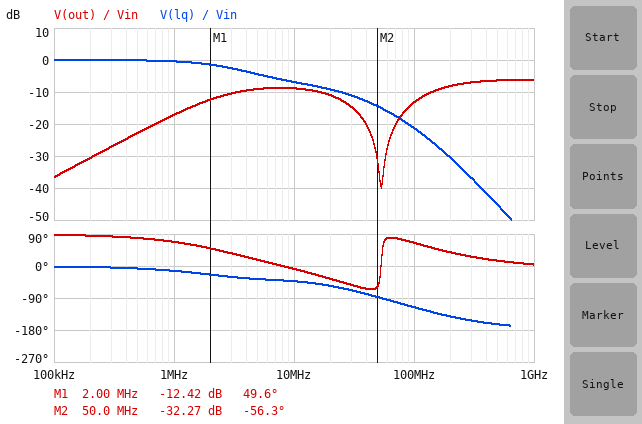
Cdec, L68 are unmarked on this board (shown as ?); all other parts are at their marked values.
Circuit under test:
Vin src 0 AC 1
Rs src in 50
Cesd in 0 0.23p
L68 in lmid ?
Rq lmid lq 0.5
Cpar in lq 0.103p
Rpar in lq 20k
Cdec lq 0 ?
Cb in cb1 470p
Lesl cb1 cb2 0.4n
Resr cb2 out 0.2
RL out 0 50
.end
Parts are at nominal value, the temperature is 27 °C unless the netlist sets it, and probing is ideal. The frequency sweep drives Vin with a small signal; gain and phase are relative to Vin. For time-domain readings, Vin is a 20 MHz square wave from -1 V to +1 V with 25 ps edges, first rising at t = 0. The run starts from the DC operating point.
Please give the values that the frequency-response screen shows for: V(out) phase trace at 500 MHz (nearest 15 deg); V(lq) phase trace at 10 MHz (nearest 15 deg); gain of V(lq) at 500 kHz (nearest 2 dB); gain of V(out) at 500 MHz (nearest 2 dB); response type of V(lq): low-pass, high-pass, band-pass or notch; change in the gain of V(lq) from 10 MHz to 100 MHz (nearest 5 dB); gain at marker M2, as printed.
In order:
15 deg
-45 deg
0 dB
-6 dB
low-pass
-15 dB
-32.27 dB
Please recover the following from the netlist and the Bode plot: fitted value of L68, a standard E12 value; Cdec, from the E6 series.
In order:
27 nH
330 pF
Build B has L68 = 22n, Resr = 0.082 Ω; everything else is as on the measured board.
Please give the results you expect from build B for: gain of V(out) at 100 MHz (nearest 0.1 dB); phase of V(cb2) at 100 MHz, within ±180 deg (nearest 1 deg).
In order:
-15.5 dB
71 deg
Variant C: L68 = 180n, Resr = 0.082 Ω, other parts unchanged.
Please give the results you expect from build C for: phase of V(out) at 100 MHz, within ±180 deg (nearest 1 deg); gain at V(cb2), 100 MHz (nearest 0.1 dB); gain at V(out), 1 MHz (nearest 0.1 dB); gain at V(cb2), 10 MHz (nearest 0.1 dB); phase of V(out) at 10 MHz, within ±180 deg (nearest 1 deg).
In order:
15 deg
-6.2 dB
-17.1 dB
-9.6 dB
-13 deg
